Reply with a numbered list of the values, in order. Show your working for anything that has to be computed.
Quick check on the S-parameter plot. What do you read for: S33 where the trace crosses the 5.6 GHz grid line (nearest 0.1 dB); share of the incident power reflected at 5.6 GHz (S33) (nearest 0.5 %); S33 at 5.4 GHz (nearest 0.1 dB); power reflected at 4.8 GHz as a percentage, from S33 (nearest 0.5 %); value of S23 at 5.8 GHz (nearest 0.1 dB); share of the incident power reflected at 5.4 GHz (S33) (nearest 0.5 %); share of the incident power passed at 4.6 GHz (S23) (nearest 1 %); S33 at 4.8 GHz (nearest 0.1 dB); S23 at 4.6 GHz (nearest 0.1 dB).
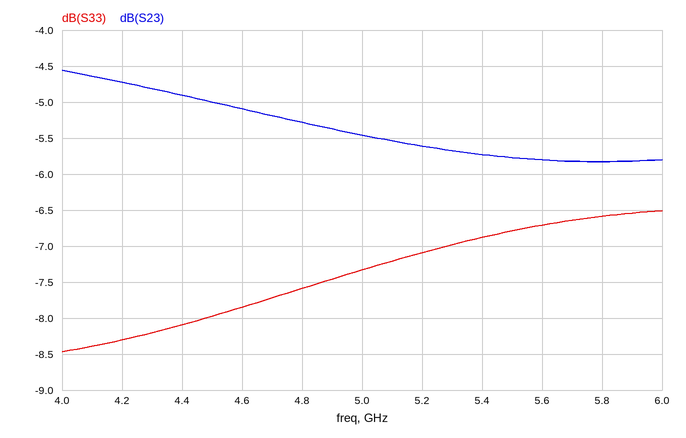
1. -6.7 dB
2. 10^(-6.7/10) ≈ 21.4 %, so 21.5 % to the nearest 0.5 %
3. -6.9 dB
4. 10^(-7.6/10) ≈ 17.4 %, so 17.5 % to the nearest 0.5 %
5. -5.8 dB
6. 10^(-6.9/10) ≈ 20.4 %, so 20.5 % to the nearest 0.5 %
7. 10^(-5.1/10) ≈ 31 %
8. -7.6 dB
9. -5.1 dB
